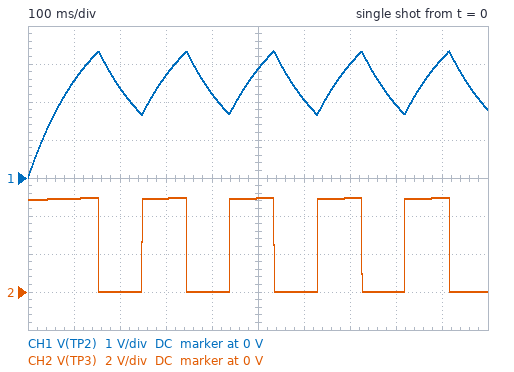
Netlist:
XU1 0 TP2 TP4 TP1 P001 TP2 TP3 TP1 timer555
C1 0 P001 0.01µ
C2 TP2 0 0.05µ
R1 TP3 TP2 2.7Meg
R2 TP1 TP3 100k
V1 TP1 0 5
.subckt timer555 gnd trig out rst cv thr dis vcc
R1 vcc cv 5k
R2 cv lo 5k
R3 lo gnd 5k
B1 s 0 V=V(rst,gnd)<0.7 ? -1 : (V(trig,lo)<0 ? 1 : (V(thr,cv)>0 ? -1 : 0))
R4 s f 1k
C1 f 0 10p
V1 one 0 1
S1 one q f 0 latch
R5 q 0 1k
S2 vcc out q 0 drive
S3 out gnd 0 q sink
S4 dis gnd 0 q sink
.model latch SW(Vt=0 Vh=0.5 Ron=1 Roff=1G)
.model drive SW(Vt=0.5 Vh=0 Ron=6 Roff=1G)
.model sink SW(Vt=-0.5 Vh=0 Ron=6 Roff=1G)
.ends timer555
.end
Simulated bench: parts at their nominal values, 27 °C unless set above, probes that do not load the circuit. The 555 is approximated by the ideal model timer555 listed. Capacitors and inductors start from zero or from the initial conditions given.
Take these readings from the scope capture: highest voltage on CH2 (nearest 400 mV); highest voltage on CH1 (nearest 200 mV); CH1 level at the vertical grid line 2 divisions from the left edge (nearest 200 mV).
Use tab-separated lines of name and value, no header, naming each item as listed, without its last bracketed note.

highest voltage on CH2	4.8 V
highest voltage on CH1	3.4 V
CH1 level at the vertical grid line 2 divisions from the left edge	2.4 V
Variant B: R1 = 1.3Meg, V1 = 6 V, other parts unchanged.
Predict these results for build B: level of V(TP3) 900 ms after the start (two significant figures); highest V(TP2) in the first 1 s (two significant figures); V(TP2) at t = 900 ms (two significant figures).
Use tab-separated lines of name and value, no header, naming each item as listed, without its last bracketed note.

level of V(TP3) 900 ms after the start	5.8 V
highest V(TP2) in the first 1 s	4.0 V
V(TP2) at t = 900 ms	3.4 V
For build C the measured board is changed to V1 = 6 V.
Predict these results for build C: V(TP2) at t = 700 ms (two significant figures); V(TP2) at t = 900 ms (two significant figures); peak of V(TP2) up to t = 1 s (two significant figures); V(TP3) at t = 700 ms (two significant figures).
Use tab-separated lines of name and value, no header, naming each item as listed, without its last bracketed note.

V(TP2) at t = 700 ms	3.6 V
V(TP2) at t = 900 ms	3.8 V
peak of V(TP2) up to t = 1 s	4.0 V
V(TP3) at t = 700 ms	5.9 V
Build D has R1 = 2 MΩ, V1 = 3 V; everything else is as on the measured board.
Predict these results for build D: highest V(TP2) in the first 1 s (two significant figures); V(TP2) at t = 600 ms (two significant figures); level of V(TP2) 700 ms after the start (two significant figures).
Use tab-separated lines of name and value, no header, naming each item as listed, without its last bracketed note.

highest V(TP2) in the first 1 s	2.0 V
V(TP2) at t = 600 ms	1.1 V
level of V(TP2) 700 ms after the start	1.7 V
